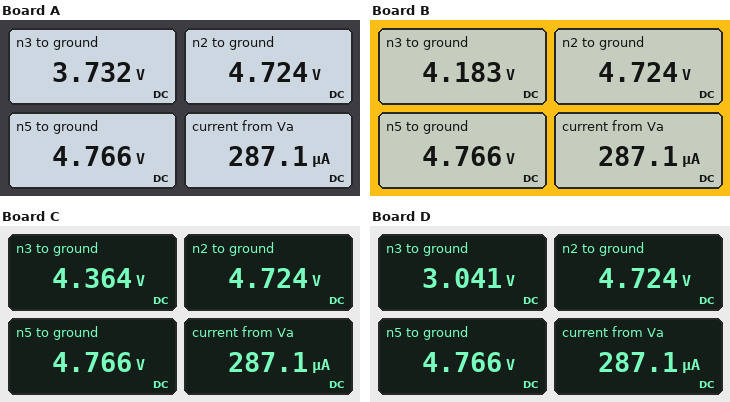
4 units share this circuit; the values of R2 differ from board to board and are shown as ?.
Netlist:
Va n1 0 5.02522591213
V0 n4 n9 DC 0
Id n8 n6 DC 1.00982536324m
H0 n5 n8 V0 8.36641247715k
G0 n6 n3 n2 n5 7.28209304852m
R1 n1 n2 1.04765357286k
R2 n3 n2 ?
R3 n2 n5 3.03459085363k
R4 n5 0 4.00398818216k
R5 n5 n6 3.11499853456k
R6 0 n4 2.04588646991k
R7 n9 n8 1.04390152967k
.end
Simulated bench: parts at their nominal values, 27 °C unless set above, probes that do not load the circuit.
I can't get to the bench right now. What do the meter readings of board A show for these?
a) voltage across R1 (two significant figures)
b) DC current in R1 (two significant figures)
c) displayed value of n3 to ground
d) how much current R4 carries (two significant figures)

300 mV
290 µA
3.732 V
1.2 mA
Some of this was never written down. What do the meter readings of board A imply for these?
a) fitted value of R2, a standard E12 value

3.3 kΩ
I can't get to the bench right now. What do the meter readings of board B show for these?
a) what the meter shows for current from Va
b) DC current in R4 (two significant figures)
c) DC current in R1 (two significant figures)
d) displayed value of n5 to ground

287.1 µA
1.2 mA
290 µA
4.766 V
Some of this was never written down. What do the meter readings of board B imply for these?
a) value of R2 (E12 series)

1.8 kΩ
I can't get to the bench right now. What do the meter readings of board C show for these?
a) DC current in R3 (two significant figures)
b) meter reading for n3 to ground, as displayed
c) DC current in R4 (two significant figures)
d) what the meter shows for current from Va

14 µA
4.364 V
1.2 mA
287.1 µA
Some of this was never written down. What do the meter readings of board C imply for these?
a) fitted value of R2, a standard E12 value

1.2 kΩ
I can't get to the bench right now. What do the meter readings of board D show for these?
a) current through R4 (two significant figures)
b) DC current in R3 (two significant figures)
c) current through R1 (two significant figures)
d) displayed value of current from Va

1.2 mA
14 µA
290 µA
287.1 µA
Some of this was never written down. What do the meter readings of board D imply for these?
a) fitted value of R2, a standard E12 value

5.6 kΩ
